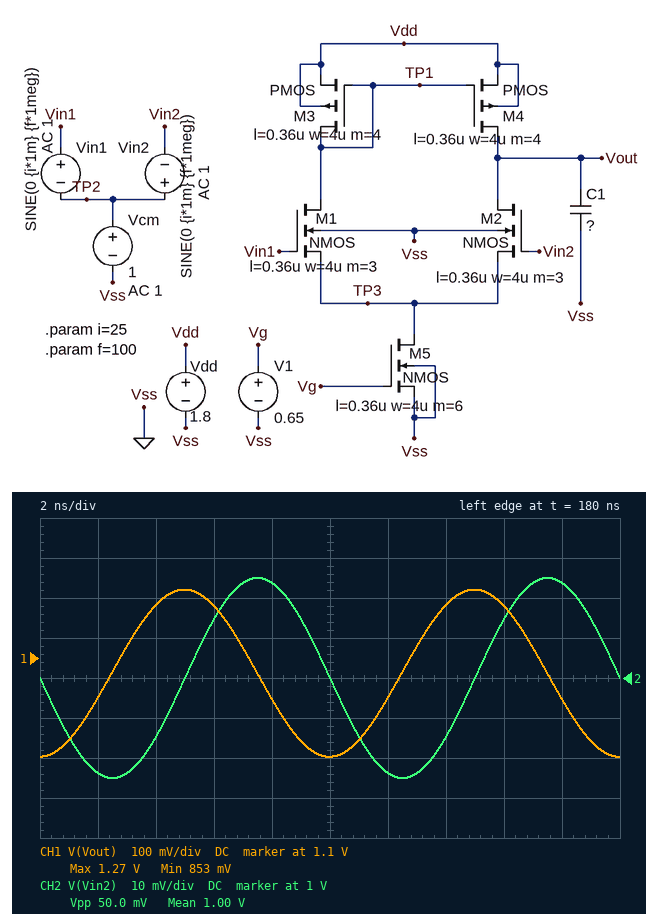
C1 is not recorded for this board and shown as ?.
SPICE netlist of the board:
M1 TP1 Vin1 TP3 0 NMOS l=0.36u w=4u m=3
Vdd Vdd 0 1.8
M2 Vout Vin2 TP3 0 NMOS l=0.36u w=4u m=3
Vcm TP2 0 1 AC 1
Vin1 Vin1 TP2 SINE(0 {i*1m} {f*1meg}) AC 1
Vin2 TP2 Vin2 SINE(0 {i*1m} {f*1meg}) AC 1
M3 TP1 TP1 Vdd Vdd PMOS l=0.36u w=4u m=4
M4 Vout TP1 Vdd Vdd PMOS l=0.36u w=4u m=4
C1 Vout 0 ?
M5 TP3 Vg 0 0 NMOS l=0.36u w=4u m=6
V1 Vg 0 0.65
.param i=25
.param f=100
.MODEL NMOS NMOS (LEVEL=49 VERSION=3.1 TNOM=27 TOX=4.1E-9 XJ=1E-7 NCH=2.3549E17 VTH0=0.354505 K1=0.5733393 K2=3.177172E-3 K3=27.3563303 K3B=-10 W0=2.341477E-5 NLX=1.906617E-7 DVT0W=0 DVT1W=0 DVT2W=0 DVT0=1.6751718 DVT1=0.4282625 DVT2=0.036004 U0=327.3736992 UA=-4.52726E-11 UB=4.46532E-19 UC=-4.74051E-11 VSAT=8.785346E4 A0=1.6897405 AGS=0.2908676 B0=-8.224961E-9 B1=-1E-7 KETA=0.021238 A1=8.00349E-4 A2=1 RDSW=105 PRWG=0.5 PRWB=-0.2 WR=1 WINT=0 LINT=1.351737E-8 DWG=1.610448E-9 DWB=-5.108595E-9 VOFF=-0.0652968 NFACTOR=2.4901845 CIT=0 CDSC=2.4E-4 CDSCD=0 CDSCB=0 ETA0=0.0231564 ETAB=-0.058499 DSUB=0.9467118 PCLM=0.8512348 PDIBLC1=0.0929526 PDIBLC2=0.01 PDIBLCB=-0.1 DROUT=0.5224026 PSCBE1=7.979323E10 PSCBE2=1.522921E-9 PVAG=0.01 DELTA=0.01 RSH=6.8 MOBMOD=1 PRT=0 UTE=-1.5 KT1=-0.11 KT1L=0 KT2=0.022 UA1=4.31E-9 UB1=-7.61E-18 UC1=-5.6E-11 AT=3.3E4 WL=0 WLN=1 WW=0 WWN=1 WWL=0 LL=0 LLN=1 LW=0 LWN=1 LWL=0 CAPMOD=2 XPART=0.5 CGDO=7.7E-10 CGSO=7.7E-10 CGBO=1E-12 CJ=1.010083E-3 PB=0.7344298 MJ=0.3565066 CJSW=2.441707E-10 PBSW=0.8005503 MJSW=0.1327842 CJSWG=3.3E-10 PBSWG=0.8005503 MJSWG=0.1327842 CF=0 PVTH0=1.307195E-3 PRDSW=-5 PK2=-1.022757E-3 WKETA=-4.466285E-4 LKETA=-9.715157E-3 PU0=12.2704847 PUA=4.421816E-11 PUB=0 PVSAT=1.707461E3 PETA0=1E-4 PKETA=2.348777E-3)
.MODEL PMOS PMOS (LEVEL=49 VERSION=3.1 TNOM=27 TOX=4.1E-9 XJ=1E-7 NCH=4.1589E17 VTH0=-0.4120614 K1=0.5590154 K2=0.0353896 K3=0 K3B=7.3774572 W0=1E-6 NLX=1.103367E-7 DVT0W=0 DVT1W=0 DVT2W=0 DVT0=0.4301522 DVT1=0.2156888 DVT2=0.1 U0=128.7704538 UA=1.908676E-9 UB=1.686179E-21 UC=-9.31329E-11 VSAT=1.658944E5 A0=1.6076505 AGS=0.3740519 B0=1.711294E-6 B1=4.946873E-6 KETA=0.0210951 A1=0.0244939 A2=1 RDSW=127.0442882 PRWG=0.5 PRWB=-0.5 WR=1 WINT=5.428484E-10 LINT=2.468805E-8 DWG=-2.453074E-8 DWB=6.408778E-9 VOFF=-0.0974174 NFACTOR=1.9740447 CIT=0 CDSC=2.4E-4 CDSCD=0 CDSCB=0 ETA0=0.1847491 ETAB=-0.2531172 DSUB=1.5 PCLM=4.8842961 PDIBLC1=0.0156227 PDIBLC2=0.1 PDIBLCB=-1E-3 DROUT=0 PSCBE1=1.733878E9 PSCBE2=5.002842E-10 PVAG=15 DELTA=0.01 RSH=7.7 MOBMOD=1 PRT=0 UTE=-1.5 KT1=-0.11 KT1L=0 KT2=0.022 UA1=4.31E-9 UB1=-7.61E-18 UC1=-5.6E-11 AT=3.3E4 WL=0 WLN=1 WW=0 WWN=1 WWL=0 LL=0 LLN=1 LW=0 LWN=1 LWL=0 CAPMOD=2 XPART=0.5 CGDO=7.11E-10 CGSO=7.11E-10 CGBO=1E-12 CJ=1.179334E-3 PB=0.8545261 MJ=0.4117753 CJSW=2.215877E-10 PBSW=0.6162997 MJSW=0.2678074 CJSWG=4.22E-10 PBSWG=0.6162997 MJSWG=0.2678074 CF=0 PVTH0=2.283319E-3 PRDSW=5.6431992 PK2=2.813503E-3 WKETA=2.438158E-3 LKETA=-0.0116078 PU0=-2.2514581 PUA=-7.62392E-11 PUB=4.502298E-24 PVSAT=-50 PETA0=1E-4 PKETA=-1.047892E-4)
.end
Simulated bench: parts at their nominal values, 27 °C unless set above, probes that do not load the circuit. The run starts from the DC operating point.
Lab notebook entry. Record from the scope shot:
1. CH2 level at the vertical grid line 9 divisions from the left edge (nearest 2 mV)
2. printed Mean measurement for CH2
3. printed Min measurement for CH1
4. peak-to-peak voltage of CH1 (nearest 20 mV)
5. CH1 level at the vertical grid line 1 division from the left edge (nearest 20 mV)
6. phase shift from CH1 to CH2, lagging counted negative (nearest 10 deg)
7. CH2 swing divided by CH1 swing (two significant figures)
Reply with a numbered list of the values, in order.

1. 1.024 V
2. 1.00 V
3. 853 mV
4. 420 mV
5. 1.00 V
6. -90 deg
7. 0.12
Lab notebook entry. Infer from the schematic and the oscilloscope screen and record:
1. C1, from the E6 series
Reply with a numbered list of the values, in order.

1. 470 fF
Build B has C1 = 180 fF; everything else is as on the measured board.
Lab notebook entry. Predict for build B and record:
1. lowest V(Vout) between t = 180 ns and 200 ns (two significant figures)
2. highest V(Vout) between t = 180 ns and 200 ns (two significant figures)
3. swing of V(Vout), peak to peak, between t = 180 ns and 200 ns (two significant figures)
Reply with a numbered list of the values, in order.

1. 580 mV
2. 1.5 V
3. 960 mV
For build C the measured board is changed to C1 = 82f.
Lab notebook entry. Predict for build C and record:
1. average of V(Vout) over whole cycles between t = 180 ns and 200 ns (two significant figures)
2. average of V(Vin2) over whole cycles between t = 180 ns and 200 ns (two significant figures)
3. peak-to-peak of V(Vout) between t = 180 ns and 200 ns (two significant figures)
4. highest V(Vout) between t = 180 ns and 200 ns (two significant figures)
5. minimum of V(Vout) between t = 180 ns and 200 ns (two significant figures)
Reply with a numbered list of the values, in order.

1. 1.0 V
2. 1.0 V
3. 1.3 V
4. 1.7 V
5. 360 mV
